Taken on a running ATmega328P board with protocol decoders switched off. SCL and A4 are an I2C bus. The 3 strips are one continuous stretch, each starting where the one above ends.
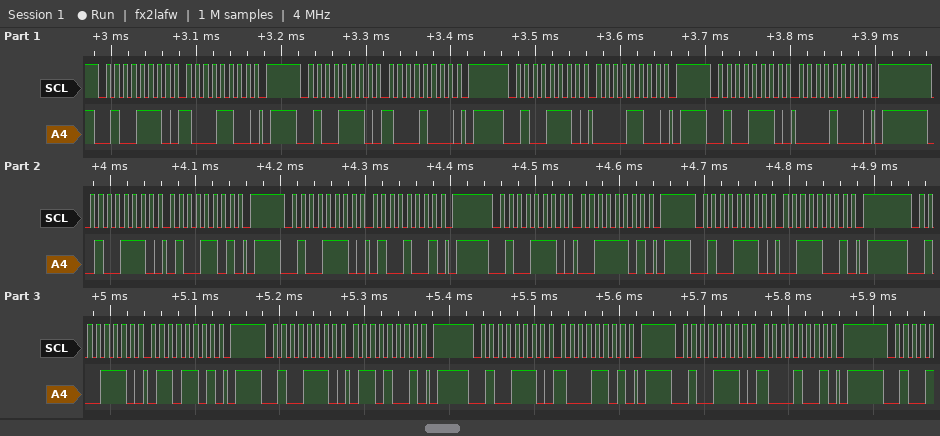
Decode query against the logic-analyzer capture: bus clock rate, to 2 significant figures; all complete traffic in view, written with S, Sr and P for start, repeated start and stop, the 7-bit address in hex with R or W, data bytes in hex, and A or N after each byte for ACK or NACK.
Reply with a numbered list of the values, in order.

1. 100 kHz
2. S 27W A 8C A P S 27W A 88 A P S 27W A 0C A P S 27W A 08 A P S 27W A 4D A P S 27W A 49 A P S 27W A 3D A P S 27W A 39 A P S 27W A 6D A P S 27W A 69 A P S 27W A 8D A P S 27W A 89 A P
